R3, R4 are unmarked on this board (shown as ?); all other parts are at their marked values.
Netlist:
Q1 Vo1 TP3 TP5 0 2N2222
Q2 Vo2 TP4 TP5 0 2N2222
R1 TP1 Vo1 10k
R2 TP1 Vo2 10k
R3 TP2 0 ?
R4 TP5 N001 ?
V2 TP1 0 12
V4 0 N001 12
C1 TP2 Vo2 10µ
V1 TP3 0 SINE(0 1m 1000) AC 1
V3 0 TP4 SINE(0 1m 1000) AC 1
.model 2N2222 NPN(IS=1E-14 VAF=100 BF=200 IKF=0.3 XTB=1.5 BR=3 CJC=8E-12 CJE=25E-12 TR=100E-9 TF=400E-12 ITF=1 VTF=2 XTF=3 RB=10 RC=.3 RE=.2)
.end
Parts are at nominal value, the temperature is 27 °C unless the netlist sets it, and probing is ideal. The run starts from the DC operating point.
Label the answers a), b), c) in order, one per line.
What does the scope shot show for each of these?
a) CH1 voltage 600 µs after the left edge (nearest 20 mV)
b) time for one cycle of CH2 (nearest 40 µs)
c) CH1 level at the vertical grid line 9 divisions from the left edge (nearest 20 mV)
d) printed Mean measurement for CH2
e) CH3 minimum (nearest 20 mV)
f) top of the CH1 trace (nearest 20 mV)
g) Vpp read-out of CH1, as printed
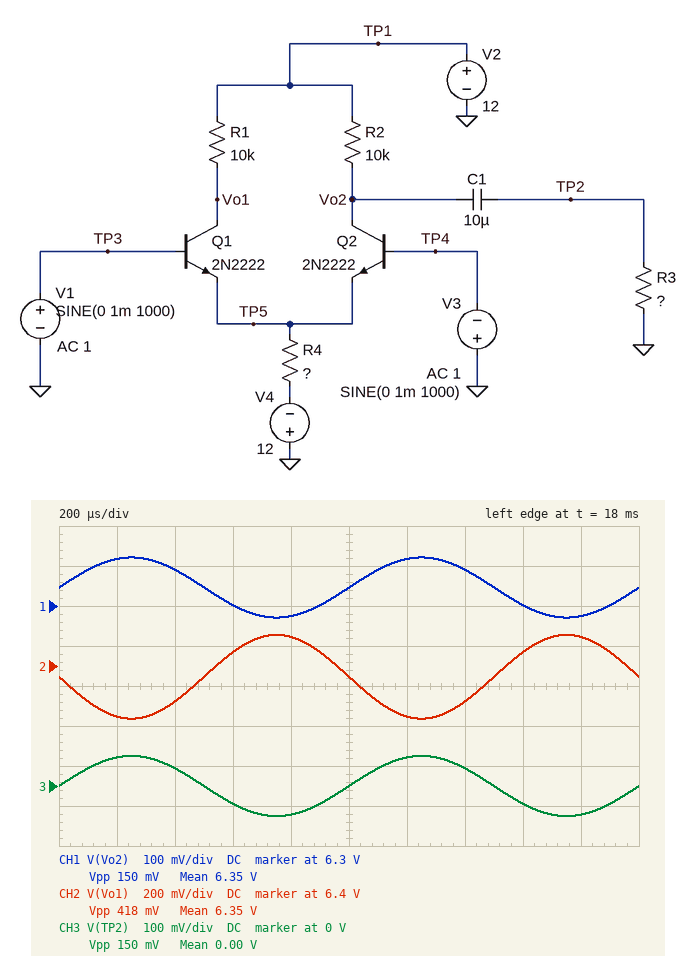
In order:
a) 6.30 V
b) 1.00 ms
c) 6.28 V
d) 6.35 V
e) -80 mV
f) 6.42 V
g) 150 mV
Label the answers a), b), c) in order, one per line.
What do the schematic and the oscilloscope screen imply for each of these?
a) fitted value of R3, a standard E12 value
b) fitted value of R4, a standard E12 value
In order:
a) 5.6 kΩ
b) 10 kΩ
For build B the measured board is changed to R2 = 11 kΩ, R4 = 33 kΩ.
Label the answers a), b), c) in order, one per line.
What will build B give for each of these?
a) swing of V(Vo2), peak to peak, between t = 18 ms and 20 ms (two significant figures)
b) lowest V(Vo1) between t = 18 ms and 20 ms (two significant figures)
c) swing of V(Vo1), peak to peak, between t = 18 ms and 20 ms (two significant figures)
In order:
a) 49 mV
b) 10 V
c) 130 mV
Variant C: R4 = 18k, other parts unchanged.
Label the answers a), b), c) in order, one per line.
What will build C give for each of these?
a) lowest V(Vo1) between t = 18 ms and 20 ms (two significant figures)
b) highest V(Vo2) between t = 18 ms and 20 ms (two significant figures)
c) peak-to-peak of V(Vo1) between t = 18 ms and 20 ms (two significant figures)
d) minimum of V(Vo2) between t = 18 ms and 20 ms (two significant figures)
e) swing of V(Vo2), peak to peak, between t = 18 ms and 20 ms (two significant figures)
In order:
a) 8.7 V
b) 8.9 V
c) 240 mV
d) 8.8 V
e) 85 mV
